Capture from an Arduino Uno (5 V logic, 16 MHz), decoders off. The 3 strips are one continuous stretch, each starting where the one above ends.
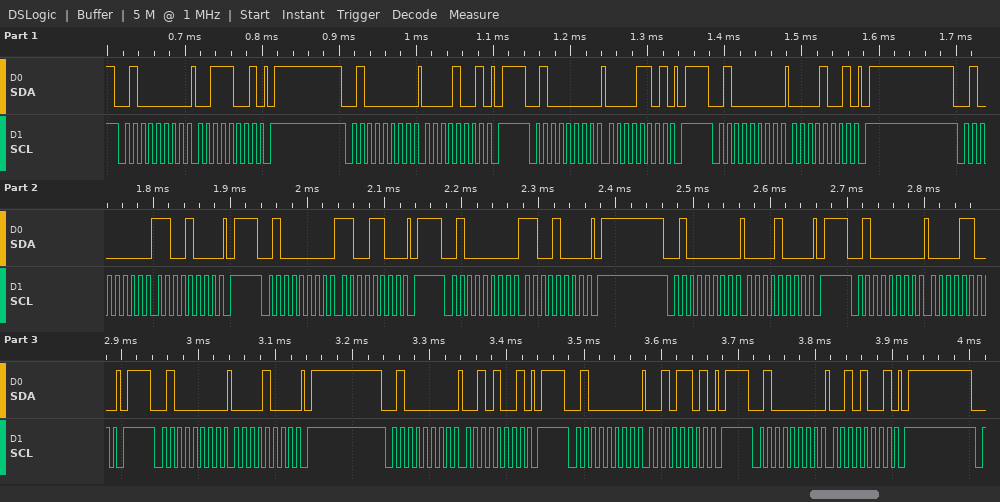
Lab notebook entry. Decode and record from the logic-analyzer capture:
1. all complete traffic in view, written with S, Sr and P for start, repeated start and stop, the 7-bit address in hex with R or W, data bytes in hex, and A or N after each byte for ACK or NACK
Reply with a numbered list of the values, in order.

1. S 20W A 39 A P S 20W A 09 A P S 20W A 0D A P S 20W A 09 A P S 20W A C8 A P S 20W A CC A P S 20W A C8 A P S 20W A 08 A P S 20W A 0C A P S 20W A 08 A P S 20W A 29 A P S 20W A 2D A P S 20W A 29 A P
